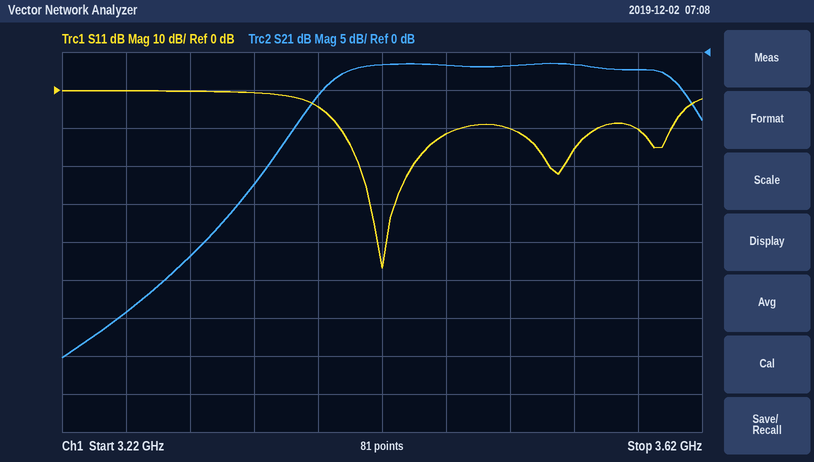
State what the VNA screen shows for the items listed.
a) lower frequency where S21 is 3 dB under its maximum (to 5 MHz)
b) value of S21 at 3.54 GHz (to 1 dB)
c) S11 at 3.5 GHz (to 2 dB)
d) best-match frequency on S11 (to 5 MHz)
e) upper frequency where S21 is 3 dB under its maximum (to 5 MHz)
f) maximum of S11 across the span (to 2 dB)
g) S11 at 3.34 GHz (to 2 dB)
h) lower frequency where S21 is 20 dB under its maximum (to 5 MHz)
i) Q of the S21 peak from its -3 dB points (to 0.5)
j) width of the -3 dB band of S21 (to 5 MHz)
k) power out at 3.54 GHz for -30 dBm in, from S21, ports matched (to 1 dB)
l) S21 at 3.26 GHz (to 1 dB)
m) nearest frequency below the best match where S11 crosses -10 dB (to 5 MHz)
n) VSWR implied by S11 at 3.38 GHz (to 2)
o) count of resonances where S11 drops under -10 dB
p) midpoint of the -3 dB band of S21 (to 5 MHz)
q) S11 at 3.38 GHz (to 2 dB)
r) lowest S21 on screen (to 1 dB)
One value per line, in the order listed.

3.385 GHz
-2 dB
-10 dB
3.420 GHz
3.605 GHz
0 dB
0 dB
3.325 GHz
16.0
220 MHz
-32 dBm
-34 dB
3.395 GHz
4
3
3.495 GHz
-4 dB
-40 dB
